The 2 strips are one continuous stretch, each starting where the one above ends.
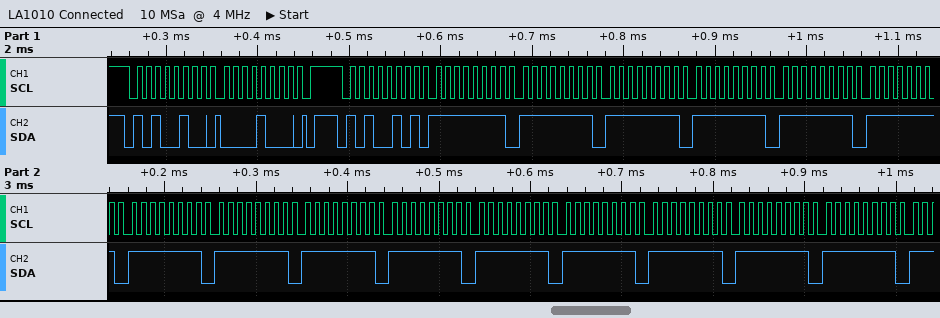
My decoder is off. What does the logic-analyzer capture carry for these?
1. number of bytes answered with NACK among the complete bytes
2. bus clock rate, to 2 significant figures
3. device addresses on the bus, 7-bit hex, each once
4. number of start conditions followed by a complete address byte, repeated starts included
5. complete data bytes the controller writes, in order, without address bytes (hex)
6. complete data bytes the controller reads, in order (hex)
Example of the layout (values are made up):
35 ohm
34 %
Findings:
0
100 kHz
0x52
2
08
FF FF FF FF FF FF FF FF FF FF FF FF FF FF FF
